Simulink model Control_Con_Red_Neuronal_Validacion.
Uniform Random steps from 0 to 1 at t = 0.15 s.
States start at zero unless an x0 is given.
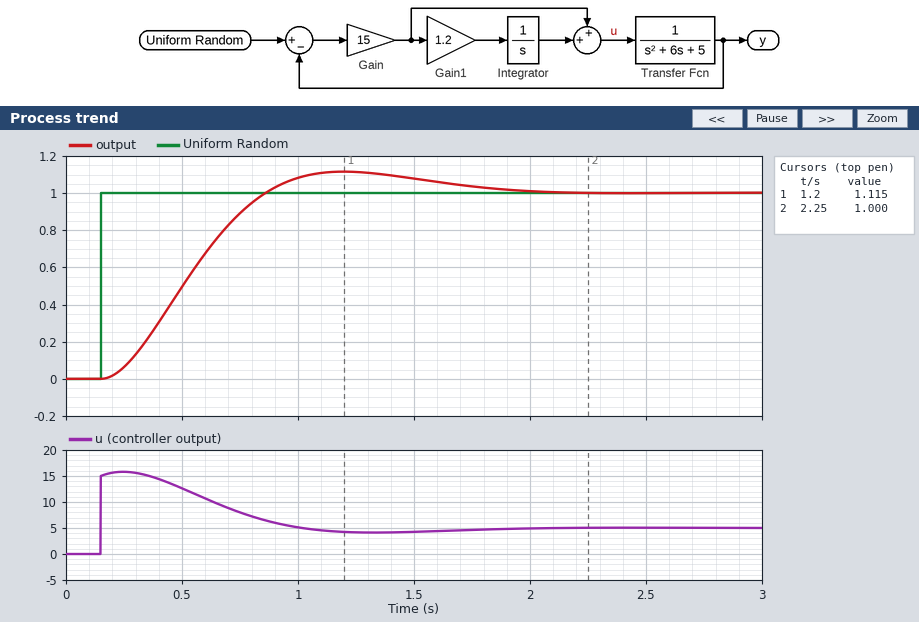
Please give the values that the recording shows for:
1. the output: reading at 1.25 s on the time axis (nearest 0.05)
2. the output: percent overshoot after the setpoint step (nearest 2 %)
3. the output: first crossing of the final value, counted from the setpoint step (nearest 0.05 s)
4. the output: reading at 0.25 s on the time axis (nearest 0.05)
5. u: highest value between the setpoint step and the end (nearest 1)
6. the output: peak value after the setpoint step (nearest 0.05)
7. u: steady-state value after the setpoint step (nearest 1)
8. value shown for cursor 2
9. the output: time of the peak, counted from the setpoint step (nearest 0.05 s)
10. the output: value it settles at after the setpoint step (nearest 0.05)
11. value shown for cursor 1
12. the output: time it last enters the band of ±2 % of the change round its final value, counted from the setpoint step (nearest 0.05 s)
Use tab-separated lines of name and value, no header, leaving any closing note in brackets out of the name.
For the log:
the output: reading at 1.25 s on the time axis	1.10
the output: percent overshoot after the setpoint step	12 %
the output: first crossing of the final value, counted from the setpoint step	0.70 s
the output: reading at 0.25 s on the time axis	0.05
u: highest value between the setpoint step and the end	16
the output: peak value after the setpoint step	1.10
u: steady-state value after the setpoint step	5
value shown for cursor 2	1.000
the output: time of the peak, counted from the setpoint step	1.05 s
the output: value it settles at after the setpoint step	1.00
value shown for cursor 1	1.115
the output: time it last enters the band of ±2 % of the change round its final value, counted from the setpoint step	1.75 s
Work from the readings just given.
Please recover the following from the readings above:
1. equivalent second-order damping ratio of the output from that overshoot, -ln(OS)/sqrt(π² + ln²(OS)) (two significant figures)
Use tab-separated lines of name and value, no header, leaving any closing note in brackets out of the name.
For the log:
equivalent second-order damping ratio of the output from that overshoot, -ln(OS)/sqrt(π² + ln²(OS))	0.56
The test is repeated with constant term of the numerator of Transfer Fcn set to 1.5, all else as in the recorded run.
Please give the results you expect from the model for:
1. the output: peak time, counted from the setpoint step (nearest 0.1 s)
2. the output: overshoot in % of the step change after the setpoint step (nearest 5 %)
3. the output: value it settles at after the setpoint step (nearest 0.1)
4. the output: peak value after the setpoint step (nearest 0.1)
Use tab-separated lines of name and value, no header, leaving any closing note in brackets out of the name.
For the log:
the output: peak time, counted from the setpoint step	0.8 s
the output: overshoot in % of the step change after the setpoint step	20 %
the output: value it settles at after the setpoint step	1.0
the output: peak value after the setpoint step	1.2
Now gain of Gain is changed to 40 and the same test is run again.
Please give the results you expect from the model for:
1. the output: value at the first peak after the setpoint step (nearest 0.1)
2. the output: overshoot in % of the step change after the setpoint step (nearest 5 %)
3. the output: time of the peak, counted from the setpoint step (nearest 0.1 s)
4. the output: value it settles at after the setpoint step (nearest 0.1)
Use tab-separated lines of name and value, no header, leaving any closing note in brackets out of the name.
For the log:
the output: value at the first peak after the setpoint step	1.3
the output: overshoot in % of the step change after the setpoint step	30 %
the output: time of the peak, counted from the setpoint step	0.5 s
the output: value it settles at after the setpoint step	1.0
